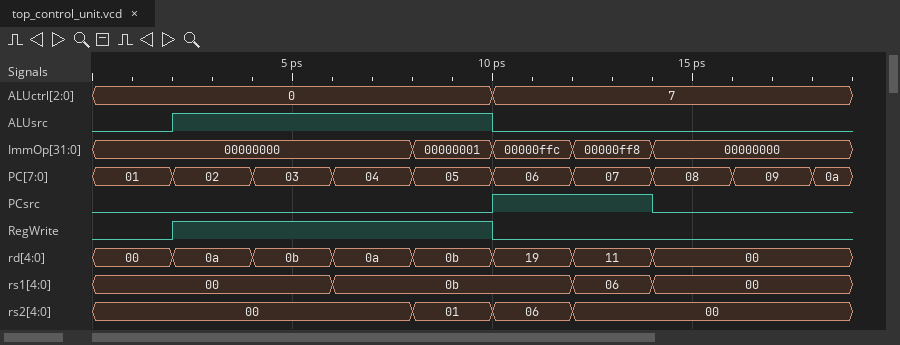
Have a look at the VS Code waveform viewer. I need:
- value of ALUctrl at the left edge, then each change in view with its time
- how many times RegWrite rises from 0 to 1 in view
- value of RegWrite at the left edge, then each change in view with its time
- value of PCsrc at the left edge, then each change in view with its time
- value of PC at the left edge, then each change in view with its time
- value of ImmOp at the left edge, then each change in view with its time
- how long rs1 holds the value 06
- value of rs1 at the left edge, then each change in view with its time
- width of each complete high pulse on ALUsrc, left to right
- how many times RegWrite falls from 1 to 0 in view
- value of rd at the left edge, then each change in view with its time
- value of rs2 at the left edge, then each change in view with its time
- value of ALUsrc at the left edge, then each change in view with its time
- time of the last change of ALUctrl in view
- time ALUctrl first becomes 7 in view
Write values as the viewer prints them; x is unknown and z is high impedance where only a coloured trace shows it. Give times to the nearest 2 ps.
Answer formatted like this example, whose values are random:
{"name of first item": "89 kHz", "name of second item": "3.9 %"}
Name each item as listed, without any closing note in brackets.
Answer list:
{"value of ALUctrl at the left edge, then each change in view with its time": "0, 7 at 10 ps", "how many times RegWrite rises from 0 to 1 in view": "1", "value of RegWrite at the left edge, then each change in view with its time": "0, 1 at 2 ps, 0 at 10 ps", "value of PCsrc at the left edge, then each change in view with its time": "0, 1 at 10 ps, 0 at 14 ps", "value of PC at the left edge, then each change in view with its time": "01, 02 at 2 ps, 03 at 4 ps, 04 at 6 ps, 05 at 8 ps, 06 at 10 ps, 07 at 12 ps, 08 at 14 ps, 09 at 16 ps, 0a at 18 ps", "value of ImmOp at the left edge, then each change in view with its time": "00000000, 00000001 at 8 ps, 00000ffc at 10 ps, 00000ff8 at 12 ps, 00000000 at 14 ps", "how long rs1 holds the value 06": "2 ps", "value of rs1 at the left edge, then each change in view with its time": "00, 0b at 6 ps, 06 at 12 ps, 00 at 14 ps", "width of each complete high pulse on ALUsrc, left to right": "8 ps", "how many times RegWrite falls from 1 to 0 in view": "1", "value of rd at the left edge, then each change in view with its time": "00, 0a at 2 ps, 0b at 4 ps, 0a at 6 ps, 0b at 8 ps, 19 at 10 ps, 11 at 12 ps, 00 at 14 ps", "value of rs2 at the left edge, then each change in view with its time": "00, 01 at 8 ps, 06 at 10 ps, 00 at 12 ps", "value of ALUsrc at the left edge, then each change in view with its time": "0, 1 at 2 ps, 0 at 10 ps", "time of the last change of ALUctrl in view": "10 ps", "time ALUctrl first becomes 7 in view": "10 ps"}
